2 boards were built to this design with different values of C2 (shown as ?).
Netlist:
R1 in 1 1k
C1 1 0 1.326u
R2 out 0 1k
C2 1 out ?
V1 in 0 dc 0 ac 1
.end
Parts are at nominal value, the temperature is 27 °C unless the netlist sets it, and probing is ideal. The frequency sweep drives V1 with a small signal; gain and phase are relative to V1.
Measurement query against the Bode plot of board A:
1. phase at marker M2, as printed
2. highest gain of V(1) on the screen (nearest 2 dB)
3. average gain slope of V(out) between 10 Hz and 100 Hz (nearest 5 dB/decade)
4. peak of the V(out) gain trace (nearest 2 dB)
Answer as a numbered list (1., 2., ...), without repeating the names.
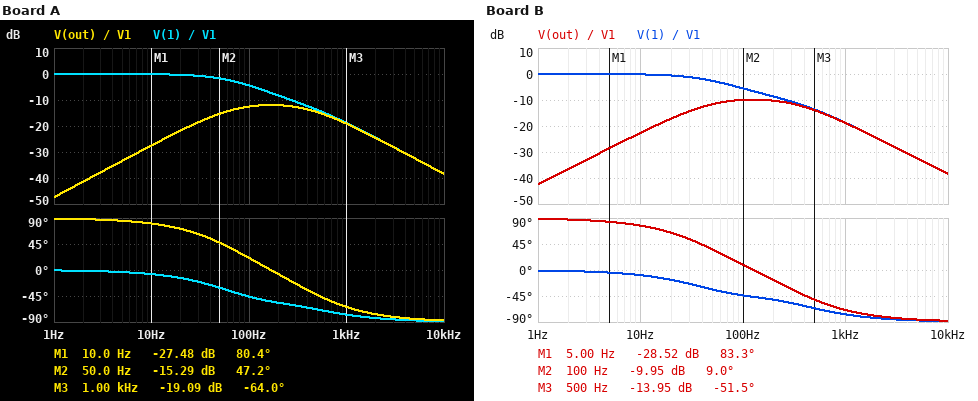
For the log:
1. 47.2 deg
2. 0 dB
3. 15 dB/decade
4. -12 dB
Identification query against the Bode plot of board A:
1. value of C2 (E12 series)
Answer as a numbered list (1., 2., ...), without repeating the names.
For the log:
1. 680 nF
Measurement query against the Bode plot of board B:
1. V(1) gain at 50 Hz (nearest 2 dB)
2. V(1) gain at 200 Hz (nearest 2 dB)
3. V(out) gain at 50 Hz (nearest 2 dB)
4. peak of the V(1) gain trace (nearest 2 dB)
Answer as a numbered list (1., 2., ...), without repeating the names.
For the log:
1. -2 dB
2. -8 dB
3. -12 dB
4. 0 dB
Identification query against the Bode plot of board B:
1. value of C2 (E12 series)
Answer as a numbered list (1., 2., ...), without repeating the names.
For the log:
1. 1.2 µF
